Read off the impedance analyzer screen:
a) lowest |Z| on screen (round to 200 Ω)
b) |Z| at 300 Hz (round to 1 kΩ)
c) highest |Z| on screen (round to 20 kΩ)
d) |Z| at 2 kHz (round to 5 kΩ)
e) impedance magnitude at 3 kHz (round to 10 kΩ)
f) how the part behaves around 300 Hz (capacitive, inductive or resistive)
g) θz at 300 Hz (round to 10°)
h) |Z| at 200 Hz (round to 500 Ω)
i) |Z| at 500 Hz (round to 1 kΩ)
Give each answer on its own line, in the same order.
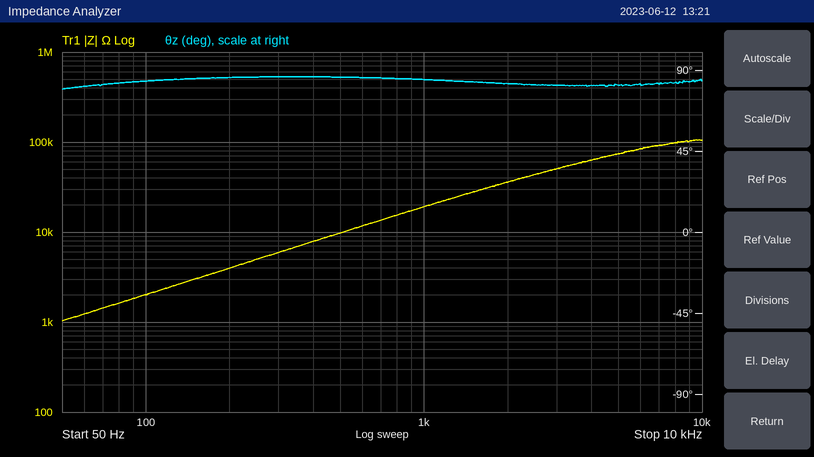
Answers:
1.0 kΩ
6 kΩ
100 kΩ
35 kΩ
50 kΩ
inductive
90°
4.0 kΩ
10 kΩ
